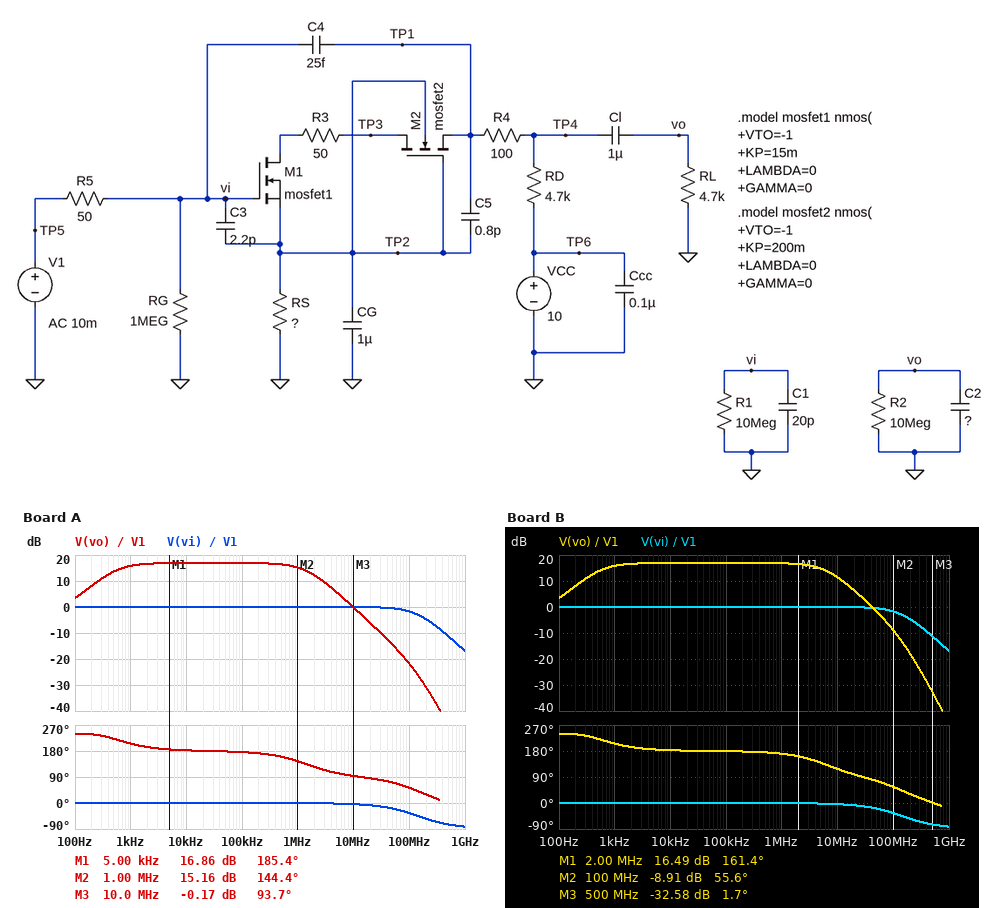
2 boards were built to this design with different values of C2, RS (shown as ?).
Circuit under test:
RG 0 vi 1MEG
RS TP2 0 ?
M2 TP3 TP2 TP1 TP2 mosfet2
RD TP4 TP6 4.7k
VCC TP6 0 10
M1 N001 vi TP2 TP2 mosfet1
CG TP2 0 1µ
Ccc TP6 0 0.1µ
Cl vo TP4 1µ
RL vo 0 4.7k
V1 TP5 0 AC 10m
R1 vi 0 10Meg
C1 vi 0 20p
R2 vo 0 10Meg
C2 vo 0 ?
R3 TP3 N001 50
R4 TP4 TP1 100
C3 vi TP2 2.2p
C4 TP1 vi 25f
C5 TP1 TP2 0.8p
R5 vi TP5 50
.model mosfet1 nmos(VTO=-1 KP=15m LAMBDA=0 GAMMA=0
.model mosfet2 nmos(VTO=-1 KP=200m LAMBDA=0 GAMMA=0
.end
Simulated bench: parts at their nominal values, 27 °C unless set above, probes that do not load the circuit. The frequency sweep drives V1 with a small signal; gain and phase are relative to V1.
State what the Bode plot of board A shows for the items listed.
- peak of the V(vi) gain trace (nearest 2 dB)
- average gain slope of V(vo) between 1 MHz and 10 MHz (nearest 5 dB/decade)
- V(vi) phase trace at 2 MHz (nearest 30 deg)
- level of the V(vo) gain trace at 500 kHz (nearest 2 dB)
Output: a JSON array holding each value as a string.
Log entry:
["0 dB", "-15 dB/decade", "0 deg", "16 dB"]
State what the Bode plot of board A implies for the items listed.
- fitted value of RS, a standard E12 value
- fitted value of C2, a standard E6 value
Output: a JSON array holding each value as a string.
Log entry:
["2.7 kΩ", "47 pF"]
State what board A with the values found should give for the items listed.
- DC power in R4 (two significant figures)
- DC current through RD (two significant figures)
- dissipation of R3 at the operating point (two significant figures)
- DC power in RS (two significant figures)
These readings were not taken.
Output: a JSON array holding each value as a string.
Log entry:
["8.8 µW", "300 µA", "4.4 µW", "240 µW"]
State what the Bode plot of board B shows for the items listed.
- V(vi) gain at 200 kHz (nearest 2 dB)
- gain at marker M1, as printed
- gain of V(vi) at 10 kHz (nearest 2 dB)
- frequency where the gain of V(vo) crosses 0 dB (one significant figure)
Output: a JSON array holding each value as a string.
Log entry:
["0 dB", "16.49 dB", "0 dB", "40 MHz"]
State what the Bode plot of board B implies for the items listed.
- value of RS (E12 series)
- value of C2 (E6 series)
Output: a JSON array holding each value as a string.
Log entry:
["2.7 kΩ", "10 pF"]
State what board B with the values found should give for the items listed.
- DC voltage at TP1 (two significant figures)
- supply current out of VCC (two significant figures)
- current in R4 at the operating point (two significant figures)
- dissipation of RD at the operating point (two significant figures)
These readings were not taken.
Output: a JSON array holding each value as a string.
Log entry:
["8.6 V", "300 µA", "300 µA", "410 µW"]
